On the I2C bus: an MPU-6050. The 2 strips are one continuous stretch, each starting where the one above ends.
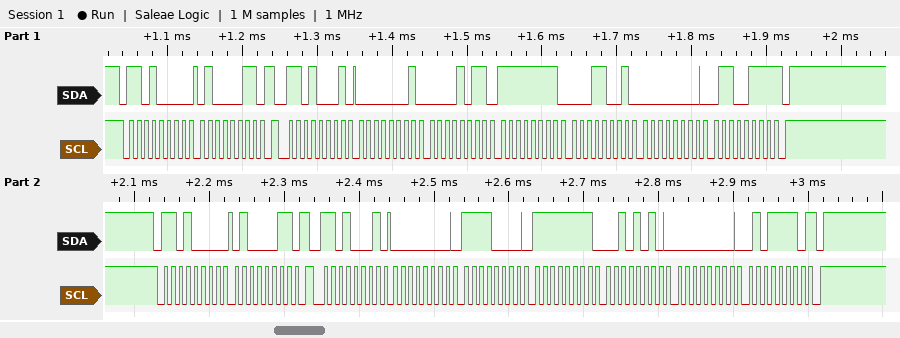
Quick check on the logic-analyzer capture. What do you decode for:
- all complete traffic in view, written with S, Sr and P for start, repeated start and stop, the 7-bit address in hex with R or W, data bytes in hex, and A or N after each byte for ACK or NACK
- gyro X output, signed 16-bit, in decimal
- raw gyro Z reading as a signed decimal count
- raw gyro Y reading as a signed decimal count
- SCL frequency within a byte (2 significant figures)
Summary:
S 68W A 43 A Sr 68R A 01 A 0B A FF A 19 A 00 A 67 N P S 68W A 43 A Sr 68R A 00 A F0 A FF A 2A A 00 A 5E N P
267
103
-231
100 kHz
